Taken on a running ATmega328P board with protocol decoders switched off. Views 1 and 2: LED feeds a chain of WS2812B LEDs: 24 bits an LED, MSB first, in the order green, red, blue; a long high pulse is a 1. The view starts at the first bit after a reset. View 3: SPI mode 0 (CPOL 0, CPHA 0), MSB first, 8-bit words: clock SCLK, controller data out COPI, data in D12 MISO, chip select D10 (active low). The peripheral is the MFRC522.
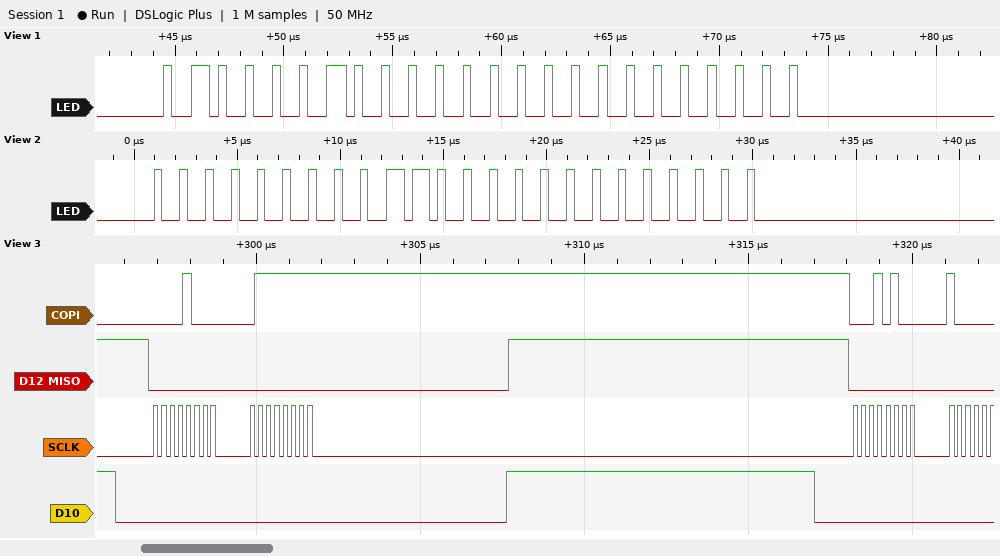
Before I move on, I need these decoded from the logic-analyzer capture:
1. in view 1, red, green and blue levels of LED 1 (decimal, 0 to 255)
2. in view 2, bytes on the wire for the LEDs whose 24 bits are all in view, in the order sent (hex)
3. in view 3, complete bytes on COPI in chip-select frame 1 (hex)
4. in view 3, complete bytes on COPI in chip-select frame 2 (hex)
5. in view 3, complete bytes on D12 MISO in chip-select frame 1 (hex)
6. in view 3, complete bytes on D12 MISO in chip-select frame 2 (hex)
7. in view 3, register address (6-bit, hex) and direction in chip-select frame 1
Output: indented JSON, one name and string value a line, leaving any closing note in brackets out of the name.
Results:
{
  "in view 1, red, green and blue levels of LED 1": "0, 66, 0",
  "in view 2, bytes on the wire for the LEDs whose 24 bits are all in view, in the order sent": "00 60 00",
  "in view 3, complete bytes on COPI in chip-select frame 1": "08 7F",
  "in view 3, complete bytes on COPI in chip-select frame 2": "14",
  "in view 3, complete bytes on D12 MISO in chip-select frame 1": "00 00",
  "in view 3, complete bytes on D12 MISO in chip-select frame 2": "00",
  "in view 3, register address (6-bit, hex) and direction in chip-select frame 1": "0x04 write"
}
